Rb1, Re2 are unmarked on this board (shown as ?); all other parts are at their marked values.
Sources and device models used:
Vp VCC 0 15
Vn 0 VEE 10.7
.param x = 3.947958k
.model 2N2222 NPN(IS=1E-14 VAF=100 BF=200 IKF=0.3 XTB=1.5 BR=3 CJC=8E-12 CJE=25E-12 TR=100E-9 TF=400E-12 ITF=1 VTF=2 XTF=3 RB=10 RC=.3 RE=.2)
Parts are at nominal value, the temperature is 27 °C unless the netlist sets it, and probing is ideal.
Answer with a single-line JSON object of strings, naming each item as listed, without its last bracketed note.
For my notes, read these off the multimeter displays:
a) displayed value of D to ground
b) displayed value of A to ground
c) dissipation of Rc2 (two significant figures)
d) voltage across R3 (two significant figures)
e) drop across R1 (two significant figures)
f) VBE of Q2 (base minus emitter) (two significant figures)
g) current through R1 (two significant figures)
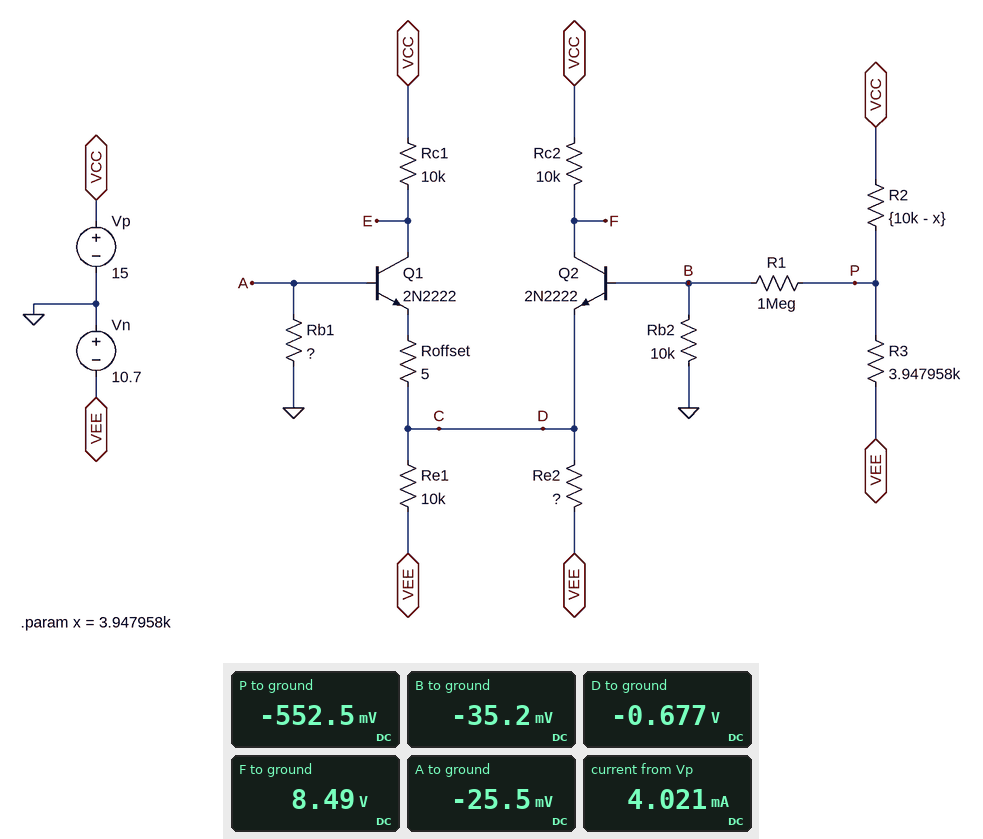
{"displayed value of D to ground": "-0.677 V", "displayed value of A to ground": "-25.5 mV", "dissipation of Rc2": "4.2 mW", "voltage across R3": "10 V", "drop across R1": "520 mV", "VBE of Q2 (base minus emitter)": "640 mV", "current through R1": "520 nA"}
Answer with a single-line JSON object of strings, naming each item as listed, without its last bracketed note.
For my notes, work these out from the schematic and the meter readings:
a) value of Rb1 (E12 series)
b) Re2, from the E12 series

{"value of Rb1": "6.8 kΩ", "Re2, from the E12 series": "22 kΩ"}
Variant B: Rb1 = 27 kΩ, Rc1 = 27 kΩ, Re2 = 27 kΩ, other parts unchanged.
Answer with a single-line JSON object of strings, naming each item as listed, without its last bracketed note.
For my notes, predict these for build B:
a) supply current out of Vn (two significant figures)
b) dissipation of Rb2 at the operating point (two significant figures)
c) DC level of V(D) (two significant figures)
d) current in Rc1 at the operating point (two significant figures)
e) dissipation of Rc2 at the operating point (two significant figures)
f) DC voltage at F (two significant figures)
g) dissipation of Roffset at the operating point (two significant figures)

{"supply current out of Vn": "3.9 mA", "dissipation of Rb2 at the operating point": "230 nW", "DC level of V(D)": "-700 mV", "current in Rc1 at the operating point": "470 µA", "dissipation of Rc2 at the operating point": "8.1 mW", "DC voltage at F": "6.0 V", "dissipation of Roffset at the operating point": "1.1 µW"}
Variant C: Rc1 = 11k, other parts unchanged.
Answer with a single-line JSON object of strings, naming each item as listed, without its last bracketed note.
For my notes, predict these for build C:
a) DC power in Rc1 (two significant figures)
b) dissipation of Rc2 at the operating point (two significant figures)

{"DC power in Rc1": "7.0 mW", "dissipation of Rc2 at the operating point": "4.3 mW"}
